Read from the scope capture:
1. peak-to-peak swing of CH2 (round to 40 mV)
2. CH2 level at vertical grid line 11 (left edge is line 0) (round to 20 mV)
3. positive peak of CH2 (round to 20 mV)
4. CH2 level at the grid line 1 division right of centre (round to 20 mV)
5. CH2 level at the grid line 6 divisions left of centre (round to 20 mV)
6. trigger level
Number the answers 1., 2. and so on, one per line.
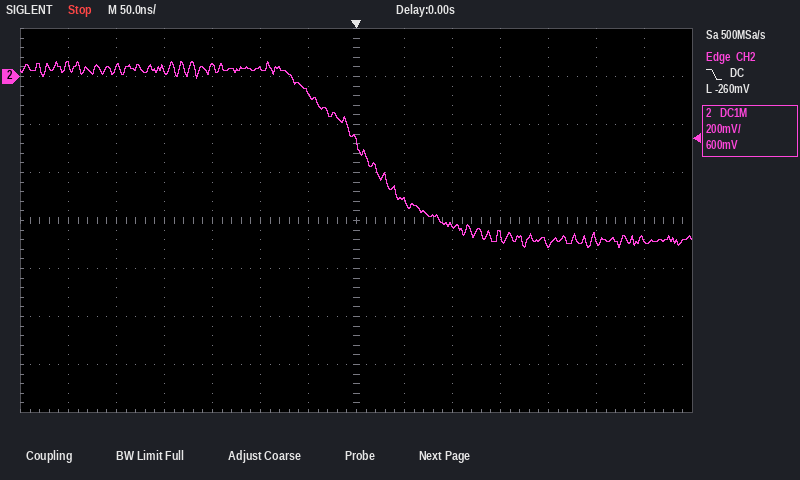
1. 760 mV
2. -700 mV
3. 60 mV
4. -520 mV
5. 40 mV
6. -260 mV
